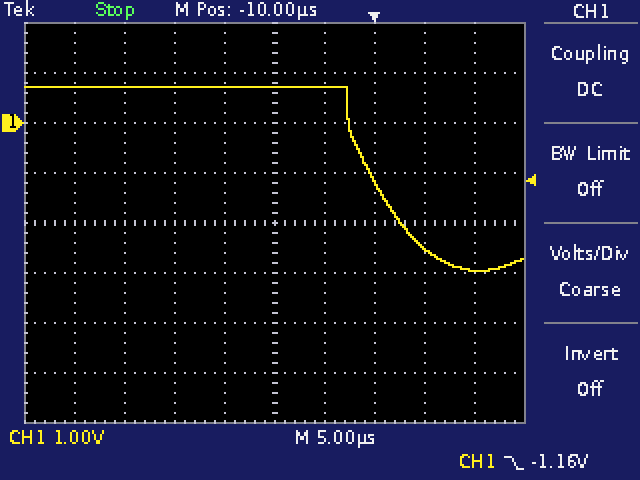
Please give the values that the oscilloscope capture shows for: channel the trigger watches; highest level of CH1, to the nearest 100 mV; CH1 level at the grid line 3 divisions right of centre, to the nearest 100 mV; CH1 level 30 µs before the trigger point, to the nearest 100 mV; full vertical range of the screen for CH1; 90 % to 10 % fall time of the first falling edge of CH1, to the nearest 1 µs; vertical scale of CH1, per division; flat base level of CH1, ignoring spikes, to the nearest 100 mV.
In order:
CH1
700 mV
-2.5 V
700 mV
8 V
8 µs
1 V
-2.9 V
